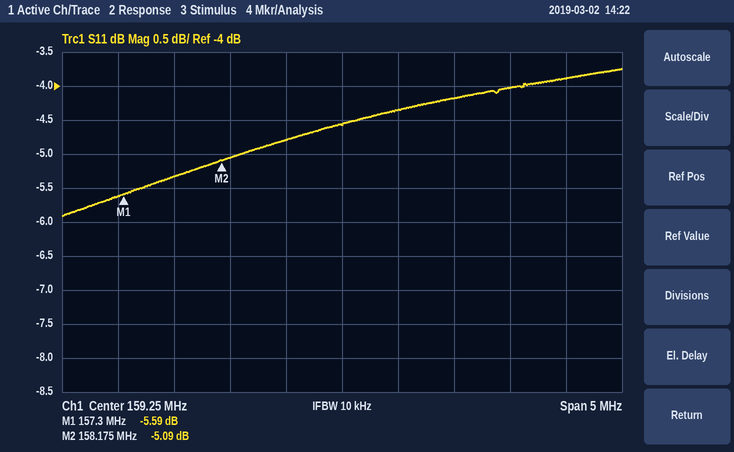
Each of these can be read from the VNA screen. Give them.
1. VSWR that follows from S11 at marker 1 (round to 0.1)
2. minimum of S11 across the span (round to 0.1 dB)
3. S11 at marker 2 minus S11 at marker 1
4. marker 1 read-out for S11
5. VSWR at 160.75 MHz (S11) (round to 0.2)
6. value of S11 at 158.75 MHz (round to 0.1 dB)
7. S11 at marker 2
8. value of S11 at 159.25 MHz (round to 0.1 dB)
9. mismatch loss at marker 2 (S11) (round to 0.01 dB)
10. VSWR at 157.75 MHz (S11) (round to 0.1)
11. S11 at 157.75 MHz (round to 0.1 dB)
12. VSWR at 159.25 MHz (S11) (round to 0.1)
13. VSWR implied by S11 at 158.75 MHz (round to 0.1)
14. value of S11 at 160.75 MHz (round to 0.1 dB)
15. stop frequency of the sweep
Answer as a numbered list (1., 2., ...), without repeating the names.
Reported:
1. 3.2
2. -5.9 dB
3. 0.50 dB
4. -5.59 dB
5. 4.4
6. -4.8 dB
7. -5.09 dB
8. -4.6 dB
9. 1.61 dB
10. 3.4
11. -5.3 dB
12. 3.9
13. 3.7
14. -4.0 dB
15. 161.75 MHz
